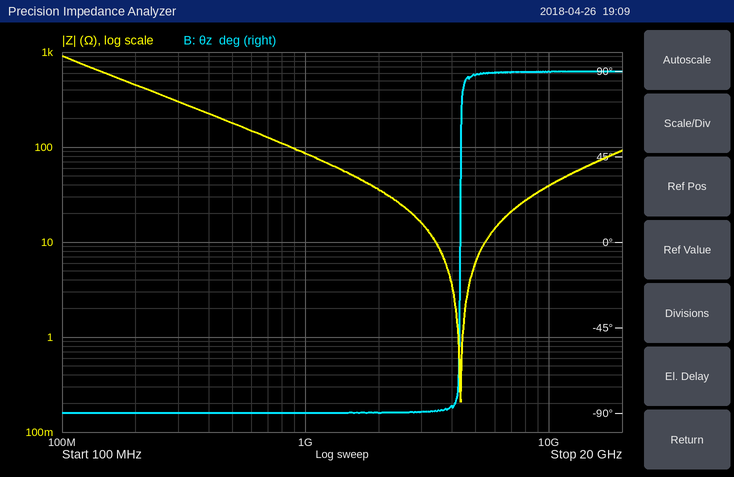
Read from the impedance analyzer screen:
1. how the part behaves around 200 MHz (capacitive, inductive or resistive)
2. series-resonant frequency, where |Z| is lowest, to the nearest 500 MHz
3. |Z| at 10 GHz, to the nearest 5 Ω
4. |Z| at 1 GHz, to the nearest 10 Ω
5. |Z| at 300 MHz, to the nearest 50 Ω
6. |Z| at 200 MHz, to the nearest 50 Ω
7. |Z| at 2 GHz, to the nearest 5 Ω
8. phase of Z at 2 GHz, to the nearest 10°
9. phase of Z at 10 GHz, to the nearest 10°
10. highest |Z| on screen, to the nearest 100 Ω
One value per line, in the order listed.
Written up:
capacitive
4.5 GHz
40 Ω
90 Ω
300 Ω
450 Ω
35 Ω
-90°
90°
900 Ω
